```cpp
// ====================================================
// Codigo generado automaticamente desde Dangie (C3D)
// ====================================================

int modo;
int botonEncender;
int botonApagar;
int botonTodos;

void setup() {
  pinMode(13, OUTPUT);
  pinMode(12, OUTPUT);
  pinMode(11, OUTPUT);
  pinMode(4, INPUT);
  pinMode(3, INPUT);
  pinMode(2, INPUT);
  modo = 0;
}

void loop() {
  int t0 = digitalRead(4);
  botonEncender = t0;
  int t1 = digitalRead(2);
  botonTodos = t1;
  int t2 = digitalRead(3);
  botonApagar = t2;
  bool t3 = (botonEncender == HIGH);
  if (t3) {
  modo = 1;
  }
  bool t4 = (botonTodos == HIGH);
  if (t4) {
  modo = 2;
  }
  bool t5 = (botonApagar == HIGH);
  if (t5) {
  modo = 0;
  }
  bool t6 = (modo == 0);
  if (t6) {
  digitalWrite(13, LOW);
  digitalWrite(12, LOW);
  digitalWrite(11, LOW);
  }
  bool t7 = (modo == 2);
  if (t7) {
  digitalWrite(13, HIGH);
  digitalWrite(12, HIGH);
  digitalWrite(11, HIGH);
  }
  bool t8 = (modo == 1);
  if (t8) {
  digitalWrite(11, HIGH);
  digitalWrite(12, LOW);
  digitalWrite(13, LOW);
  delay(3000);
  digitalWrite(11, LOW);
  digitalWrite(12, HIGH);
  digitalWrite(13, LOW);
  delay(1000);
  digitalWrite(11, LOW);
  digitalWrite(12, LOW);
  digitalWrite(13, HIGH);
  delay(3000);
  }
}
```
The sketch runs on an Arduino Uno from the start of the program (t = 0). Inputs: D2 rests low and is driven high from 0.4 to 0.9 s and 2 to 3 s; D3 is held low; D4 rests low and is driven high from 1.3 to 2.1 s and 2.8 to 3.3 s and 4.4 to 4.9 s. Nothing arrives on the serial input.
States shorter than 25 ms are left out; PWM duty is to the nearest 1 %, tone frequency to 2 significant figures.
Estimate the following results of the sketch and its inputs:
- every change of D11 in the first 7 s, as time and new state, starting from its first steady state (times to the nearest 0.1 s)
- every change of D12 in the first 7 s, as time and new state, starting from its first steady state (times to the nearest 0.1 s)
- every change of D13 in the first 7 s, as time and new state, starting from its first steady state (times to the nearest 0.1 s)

0 s low; 0.4 s high; 4.3 s low
0 s low; 0.4 s high; 1.3 s low; 4.3 s high; 5.3 s low
0 s low; 0.4 s high; 1.3 s low; 5.3 s high
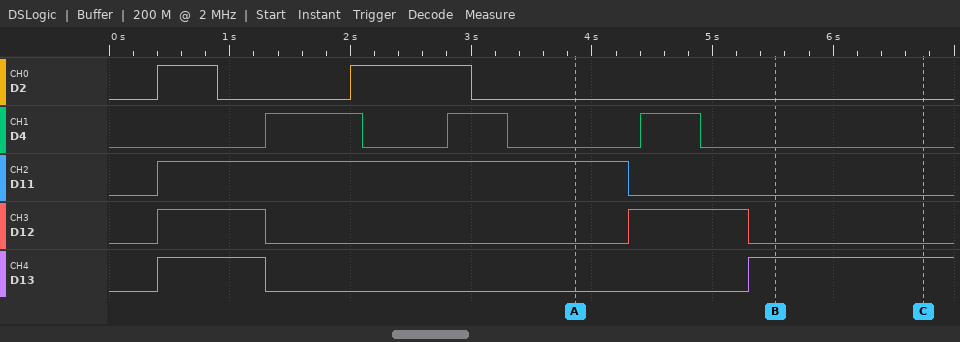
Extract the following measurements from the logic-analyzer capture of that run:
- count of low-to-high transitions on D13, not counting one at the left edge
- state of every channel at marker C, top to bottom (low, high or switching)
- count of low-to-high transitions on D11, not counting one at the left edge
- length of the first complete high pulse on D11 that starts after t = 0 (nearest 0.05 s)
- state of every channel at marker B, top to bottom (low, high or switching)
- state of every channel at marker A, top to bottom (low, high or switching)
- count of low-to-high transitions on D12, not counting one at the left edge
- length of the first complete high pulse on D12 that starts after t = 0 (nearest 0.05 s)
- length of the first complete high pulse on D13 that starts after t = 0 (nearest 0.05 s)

2
D2 low, D4 low, D11 low, D12 low, D13 high
1
3.90 s
D2 low, D4 low, D11 low, D12 low, D13 high
D2 low, D4 low, D11 high, D12 low, D13 low
2
0.90 s
0.90 s
